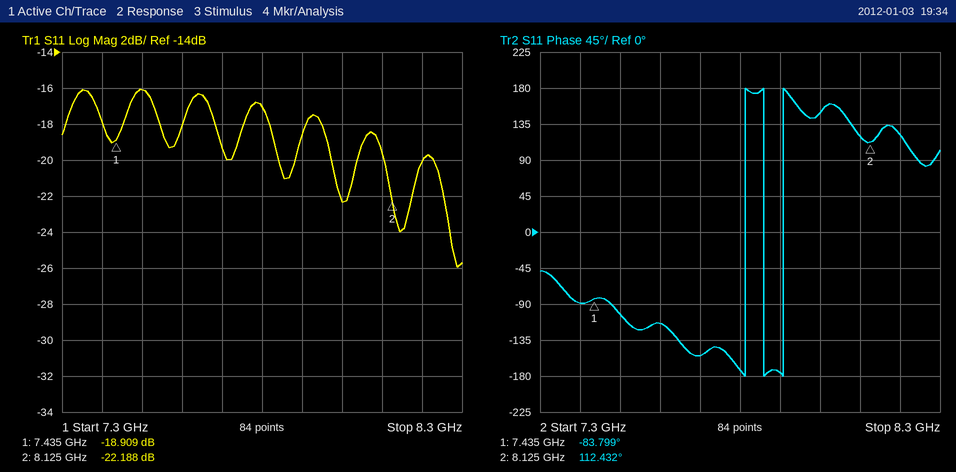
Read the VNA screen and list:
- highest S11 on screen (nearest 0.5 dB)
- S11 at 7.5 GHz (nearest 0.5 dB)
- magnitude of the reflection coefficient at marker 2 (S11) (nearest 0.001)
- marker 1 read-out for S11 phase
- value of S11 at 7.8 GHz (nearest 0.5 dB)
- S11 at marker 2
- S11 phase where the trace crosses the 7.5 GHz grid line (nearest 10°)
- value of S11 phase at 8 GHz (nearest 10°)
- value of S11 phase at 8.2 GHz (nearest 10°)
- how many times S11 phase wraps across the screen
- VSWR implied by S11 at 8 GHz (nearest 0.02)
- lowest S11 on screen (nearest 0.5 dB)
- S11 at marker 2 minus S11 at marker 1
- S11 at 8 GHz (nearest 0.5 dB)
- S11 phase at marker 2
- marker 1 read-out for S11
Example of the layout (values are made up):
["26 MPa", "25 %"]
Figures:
["-16.0 dB", "-16.0 dB", "0.078", "-83.799°", "-17.0 dB", "-22.188 dB", "-100°", "150°", "120°", "3", "1.16", "-26.0 dB", "-3.279 dB", "-22.5 dB", "112.432°", "-18.909 dB"]
